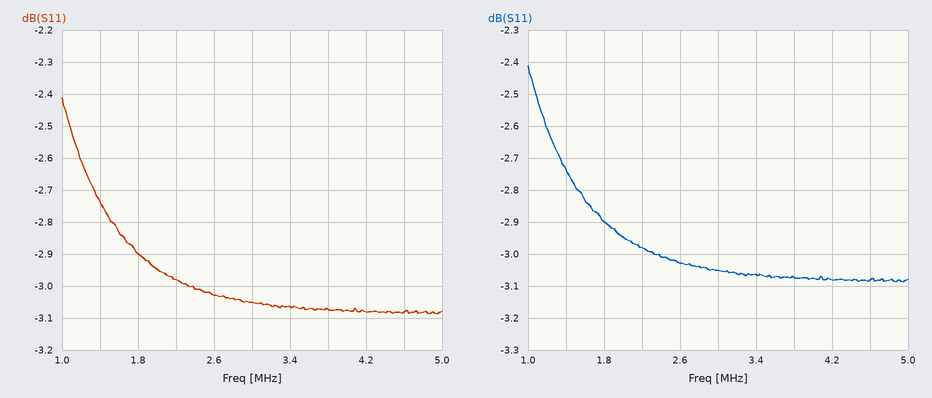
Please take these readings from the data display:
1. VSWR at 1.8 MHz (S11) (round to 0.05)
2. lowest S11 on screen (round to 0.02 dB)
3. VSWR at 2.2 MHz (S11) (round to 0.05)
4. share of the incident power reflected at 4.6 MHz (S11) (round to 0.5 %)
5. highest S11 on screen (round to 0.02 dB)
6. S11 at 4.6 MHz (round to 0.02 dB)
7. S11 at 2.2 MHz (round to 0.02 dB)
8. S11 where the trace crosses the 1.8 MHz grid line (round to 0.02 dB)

6.05
-3.08 dB
5.90
49.0 %
-2.42 dB
-3.08 dB
-2.98 dB
-2.90 dB
